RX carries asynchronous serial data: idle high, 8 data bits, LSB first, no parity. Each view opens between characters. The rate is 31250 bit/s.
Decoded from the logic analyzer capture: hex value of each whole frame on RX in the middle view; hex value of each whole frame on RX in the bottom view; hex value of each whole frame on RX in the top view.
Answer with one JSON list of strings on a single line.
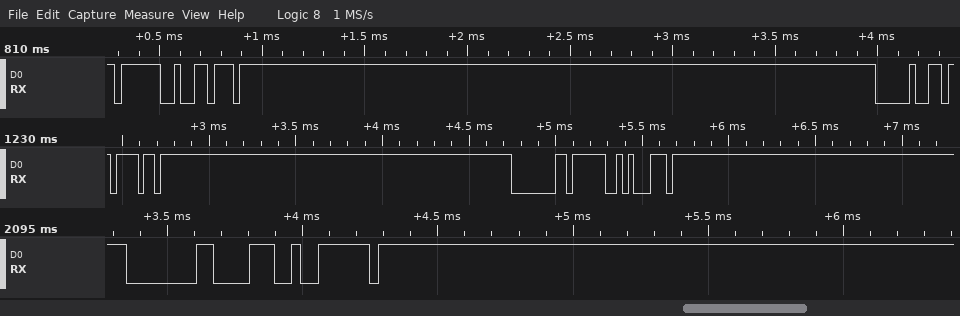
["6F, 80, 3F, 71", "80, 38, 7E", "3F, 76, 90"]
